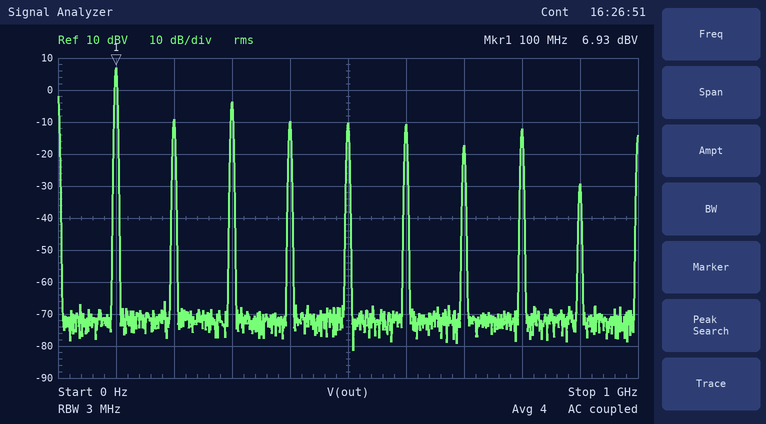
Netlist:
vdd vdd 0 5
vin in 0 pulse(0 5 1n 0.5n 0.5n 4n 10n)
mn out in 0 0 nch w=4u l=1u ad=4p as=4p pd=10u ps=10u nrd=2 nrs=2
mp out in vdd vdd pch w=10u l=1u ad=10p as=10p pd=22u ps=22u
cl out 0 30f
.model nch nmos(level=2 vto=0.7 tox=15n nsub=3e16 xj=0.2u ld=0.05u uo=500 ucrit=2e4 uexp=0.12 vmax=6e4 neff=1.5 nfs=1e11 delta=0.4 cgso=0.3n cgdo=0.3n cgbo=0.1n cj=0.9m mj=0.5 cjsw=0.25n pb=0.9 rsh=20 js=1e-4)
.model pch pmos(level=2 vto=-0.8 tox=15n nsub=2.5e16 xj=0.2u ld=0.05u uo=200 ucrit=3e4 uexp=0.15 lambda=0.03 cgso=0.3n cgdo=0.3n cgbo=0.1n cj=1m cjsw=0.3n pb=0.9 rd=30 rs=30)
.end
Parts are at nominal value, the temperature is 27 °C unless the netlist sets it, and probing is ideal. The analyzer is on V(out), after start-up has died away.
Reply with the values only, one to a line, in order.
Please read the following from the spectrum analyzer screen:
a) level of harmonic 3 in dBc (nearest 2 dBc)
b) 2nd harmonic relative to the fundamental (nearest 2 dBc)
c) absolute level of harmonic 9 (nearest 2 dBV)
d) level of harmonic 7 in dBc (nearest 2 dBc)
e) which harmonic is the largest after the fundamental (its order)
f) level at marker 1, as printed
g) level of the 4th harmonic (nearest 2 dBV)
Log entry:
-10 dBc
-16 dBc
-30 dBV
-24 dBc
3
6.93 dBV
-10 dBV
